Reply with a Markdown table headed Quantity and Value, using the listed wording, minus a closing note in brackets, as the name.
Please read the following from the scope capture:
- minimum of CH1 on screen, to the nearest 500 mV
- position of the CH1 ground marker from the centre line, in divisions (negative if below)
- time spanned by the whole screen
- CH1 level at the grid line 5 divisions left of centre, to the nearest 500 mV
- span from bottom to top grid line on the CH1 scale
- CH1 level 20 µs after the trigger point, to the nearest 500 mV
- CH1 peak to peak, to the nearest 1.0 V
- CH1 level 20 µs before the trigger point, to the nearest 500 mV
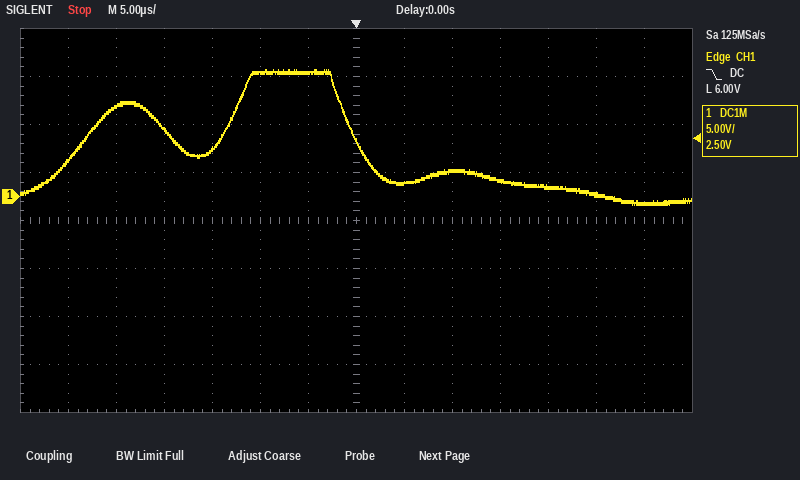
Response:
| Quantity | Value |
|---|---|
| minimum of CH1 on screen, to the nearest 500 mV | -1.0 V |
| position of the CH1 ground marker from the centre line, in divisions | +0.5 div |
| time spanned by the whole screen | 70 µs |
| CH1 level at the grid line 5 divisions left of centre, to the nearest 500 mV | 9.5 V |
| span from bottom to top grid line on the CH1 scale | 40 V |
| CH1 level 20 µs after the trigger point, to the nearest 500 mV | 1.0 V |
| CH1 peak to peak, to the nearest 1.0 V | 14.0 V |
| CH1 level 20 µs before the trigger point, to the nearest 500 mV | 7.0 V |
